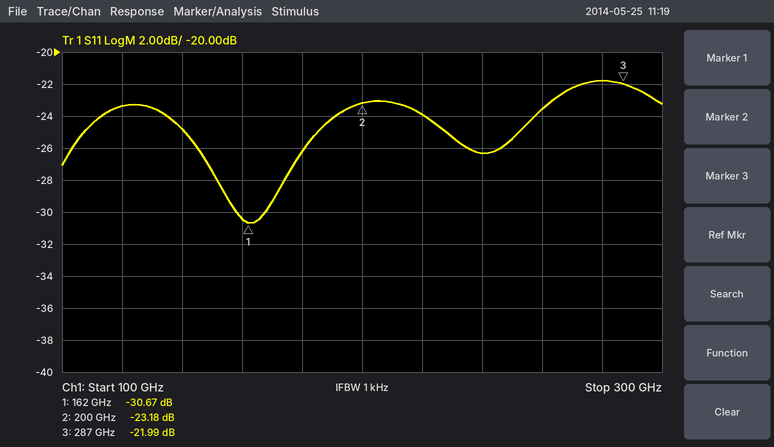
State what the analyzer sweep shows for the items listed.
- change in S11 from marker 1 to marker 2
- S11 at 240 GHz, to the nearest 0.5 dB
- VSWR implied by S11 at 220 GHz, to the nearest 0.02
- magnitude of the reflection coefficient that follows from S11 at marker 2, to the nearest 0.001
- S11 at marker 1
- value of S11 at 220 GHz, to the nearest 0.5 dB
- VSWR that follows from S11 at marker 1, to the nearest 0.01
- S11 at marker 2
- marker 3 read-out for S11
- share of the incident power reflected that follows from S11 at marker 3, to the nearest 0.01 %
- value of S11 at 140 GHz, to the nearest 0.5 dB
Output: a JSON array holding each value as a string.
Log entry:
["7.49 dB", "-26.5 dB", "1.14", "0.069", "-30.67 dB", "-24.0 dB", "1.06", "-23.18 dB", "-21.99 dB", "0.63 %", "-25.0 dB"]
